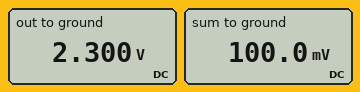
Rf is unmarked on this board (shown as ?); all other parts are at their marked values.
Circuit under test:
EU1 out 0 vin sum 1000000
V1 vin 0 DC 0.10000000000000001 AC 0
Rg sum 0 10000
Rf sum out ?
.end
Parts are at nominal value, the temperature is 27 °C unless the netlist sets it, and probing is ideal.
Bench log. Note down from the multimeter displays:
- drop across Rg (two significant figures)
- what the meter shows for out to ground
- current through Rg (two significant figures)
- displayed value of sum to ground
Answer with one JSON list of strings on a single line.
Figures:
["100 mV", "2.300 V", "10 µA", "100.0 mV"]
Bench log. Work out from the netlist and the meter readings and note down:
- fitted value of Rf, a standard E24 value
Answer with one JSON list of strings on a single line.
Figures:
["220 kΩ"]
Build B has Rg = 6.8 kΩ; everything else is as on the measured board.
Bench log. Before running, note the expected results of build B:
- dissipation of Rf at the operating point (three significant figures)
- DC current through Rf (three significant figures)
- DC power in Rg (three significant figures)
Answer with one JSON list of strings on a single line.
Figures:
["47.6 µW", "14.7 µA", "1.47 µW"]
